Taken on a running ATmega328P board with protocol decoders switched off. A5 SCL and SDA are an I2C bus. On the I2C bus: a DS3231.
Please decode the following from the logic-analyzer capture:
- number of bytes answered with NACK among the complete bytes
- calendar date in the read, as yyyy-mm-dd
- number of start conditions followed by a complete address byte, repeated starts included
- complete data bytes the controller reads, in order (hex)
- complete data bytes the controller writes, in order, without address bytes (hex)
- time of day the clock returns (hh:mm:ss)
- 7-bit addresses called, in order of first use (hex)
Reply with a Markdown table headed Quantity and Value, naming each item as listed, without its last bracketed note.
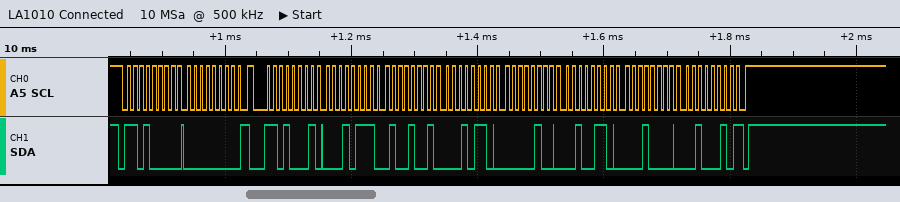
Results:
| Quantity | Value |
|---|---|
| number of bytes answered with NACK among the complete bytes | 1 |
| calendar date in the read, as yyyy-mm-dd | 2022-10-26 |
| number of start conditions followed by a complete address byte, repeated starts included | 2 |
| complete data bytes the controller reads, in order | 17 49 16 04 26 10 22 |
| complete data bytes the controller writes, in order, without address bytes | 00 |
| time of day the clock returns | 16:49:17 |
| 7-bit addresses called, in order of first use | 0x68 |
